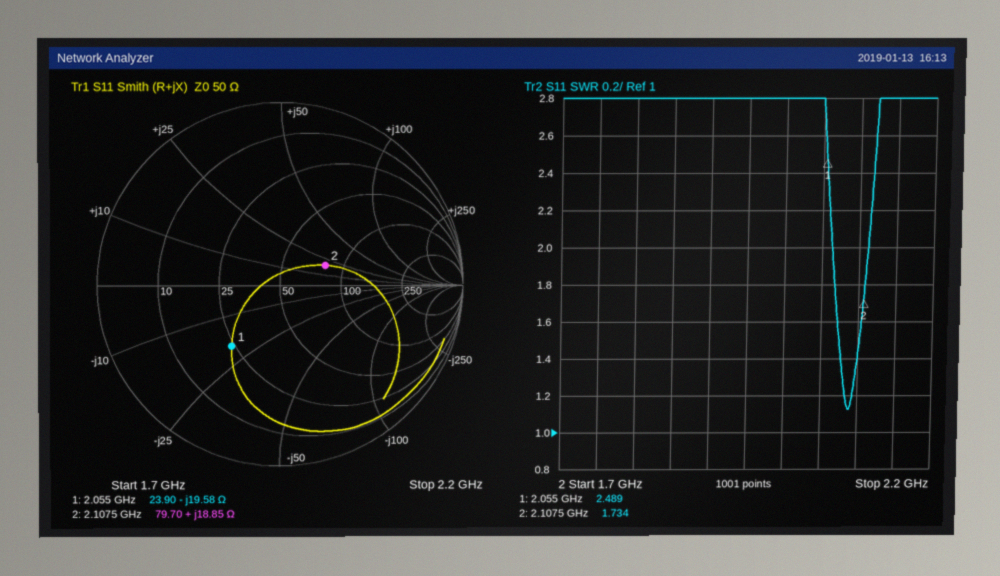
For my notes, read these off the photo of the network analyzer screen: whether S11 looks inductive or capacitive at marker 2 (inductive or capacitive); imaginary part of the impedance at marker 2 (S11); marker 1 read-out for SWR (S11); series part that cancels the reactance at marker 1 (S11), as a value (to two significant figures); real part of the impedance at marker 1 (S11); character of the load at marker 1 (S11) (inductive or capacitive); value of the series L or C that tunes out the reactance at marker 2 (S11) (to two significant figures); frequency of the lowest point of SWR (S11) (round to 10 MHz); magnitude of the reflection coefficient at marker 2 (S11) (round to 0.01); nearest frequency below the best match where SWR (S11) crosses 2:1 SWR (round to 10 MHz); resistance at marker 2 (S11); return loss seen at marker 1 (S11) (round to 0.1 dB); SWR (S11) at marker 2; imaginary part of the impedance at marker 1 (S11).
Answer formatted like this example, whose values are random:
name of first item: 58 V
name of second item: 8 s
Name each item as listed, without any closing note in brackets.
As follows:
whether S11 looks inductive or capacitive at marker 2: inductive
imaginary part of the impedance at marker 2: +18.85 Ω
marker 1 read-out for SWR: 2.489
series part that cancels the reactance at marker 1 (S11), as a value: 1.5 nH
real part of the impedance at marker 1: 23.90 Ω
character of the load at marker 1 (S11): capacitive
value of the series L or C that tunes out the reactance at marker 2 (S11): 4.0 pF
frequency of the lowest point of SWR (S11): 2.09 GHz
magnitude of the reflection coefficient at marker 2 (S11): 0.27
nearest frequency below the best match where SWR (S11) crosses 2:1 SWR: 2.06 GHz
resistance at marker 2: 79.70 Ω
return loss seen at marker 1 (S11): 7.4 dB
SWR (S11) at marker 2: 1.734
imaginary part of the impedance at marker 1: -19.58 Ω
